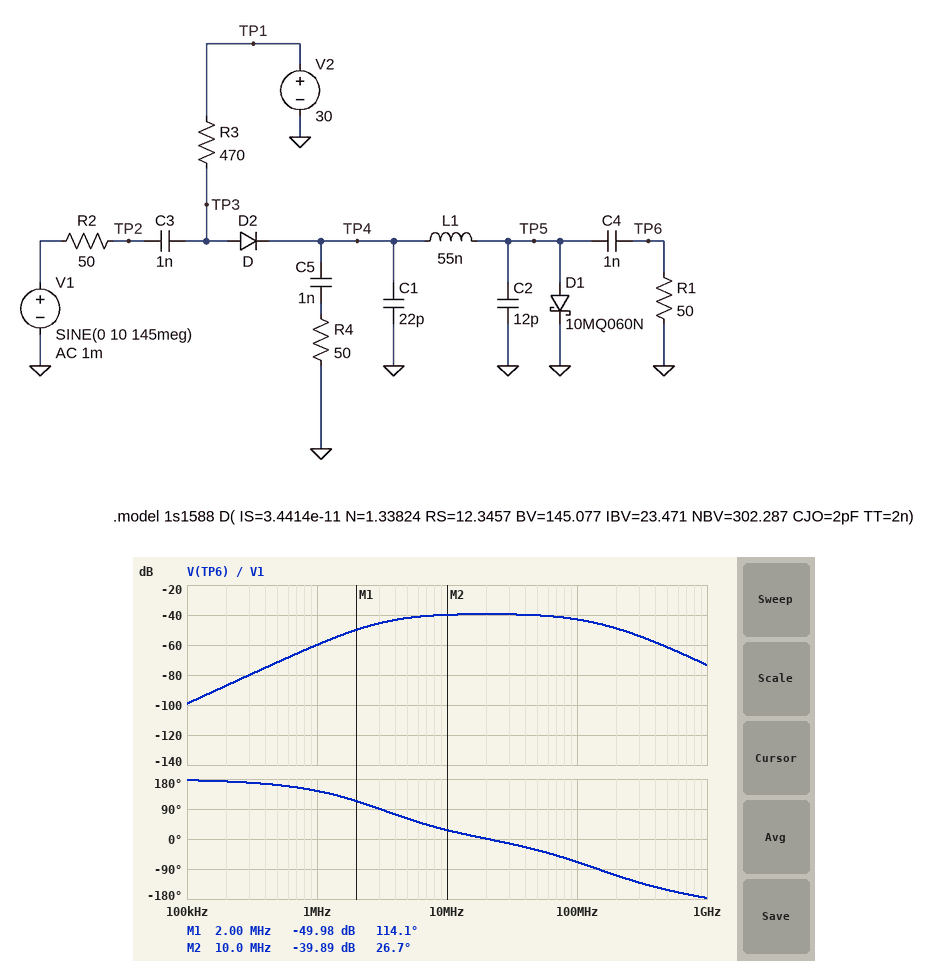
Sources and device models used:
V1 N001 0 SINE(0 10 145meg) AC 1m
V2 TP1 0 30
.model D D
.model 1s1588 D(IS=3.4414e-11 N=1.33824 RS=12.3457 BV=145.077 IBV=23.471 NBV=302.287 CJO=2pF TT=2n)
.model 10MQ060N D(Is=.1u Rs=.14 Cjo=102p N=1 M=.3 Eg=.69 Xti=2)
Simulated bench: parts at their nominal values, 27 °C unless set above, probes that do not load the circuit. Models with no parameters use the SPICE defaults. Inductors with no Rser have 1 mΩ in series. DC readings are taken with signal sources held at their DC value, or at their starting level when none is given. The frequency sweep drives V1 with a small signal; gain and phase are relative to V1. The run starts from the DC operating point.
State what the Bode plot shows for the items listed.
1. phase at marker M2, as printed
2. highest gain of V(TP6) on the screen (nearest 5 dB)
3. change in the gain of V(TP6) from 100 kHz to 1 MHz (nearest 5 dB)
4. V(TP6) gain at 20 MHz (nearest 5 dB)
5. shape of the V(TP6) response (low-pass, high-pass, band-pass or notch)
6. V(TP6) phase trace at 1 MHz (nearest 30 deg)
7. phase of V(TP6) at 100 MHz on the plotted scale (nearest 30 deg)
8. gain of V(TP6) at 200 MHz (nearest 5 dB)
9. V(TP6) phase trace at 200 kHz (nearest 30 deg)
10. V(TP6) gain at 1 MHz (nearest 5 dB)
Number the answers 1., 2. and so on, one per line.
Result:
1. 26.7 deg
2. -40 dB
3. 40 dB
4. -40 dB
5. band-pass
6. 150 deg
7. -60 deg
8. -50 dB
9. 180 deg
10. -60 dB
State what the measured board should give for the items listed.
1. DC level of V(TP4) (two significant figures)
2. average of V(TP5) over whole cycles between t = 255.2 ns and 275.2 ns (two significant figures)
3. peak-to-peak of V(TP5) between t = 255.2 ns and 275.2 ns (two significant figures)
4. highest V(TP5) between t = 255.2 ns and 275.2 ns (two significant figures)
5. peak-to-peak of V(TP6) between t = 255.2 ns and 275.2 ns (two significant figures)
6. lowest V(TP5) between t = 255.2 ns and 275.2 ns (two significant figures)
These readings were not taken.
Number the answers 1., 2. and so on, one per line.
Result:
1. 350 mV
2. 320 mV
3. 220 mV
4. 390 mV
5. 220 mV
6. 170 mV
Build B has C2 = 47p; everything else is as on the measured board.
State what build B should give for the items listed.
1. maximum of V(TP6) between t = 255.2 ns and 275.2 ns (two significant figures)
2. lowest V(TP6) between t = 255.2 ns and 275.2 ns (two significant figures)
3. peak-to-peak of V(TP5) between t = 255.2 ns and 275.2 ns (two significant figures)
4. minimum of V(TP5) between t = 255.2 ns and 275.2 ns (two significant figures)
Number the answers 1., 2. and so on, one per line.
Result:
1. 65 mV
2. -130 mV
3. 200 mV
4. 190 mV
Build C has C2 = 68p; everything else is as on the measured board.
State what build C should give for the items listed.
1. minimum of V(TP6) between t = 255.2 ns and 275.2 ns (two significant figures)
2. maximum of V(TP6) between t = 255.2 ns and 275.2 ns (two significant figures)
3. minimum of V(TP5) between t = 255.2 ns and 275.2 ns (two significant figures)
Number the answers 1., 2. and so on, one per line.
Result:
1. -120 mV
2. 63 mV
3. 200 mV
